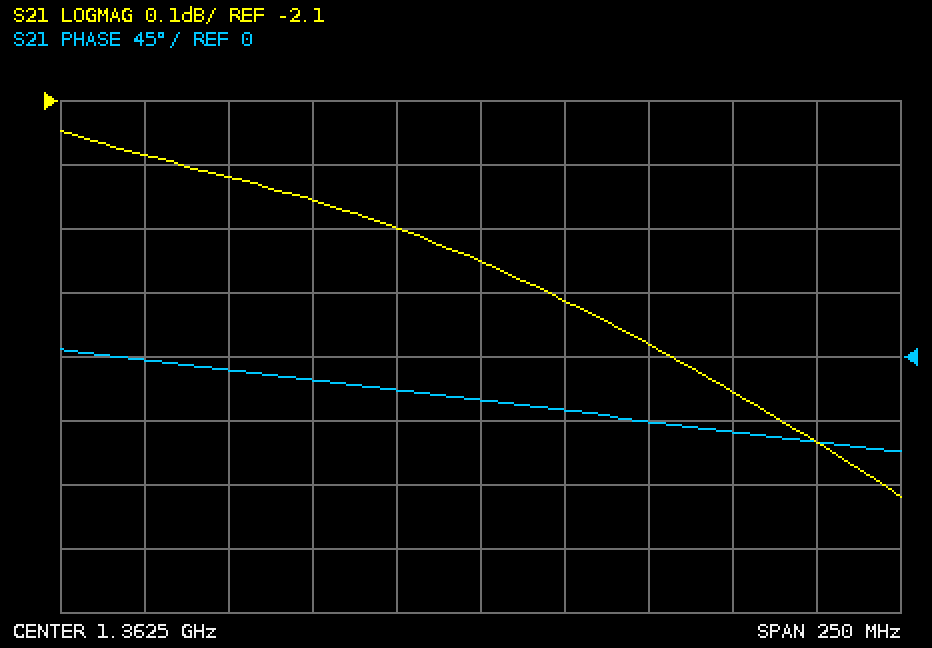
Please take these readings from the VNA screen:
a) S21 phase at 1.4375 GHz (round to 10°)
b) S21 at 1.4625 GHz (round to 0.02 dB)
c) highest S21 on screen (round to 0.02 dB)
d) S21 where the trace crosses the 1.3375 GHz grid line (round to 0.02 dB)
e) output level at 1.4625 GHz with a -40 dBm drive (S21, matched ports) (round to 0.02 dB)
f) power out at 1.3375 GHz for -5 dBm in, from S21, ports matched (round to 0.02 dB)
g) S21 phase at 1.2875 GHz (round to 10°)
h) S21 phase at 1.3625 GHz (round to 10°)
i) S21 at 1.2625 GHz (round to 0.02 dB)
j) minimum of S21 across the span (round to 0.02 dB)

-50°
-2.64 dB
-2.14 dB
-2.30 dB
-42.64 dBm
-7.30 dBm
-10°
-30°
-2.18 dB
-2.72 dB
